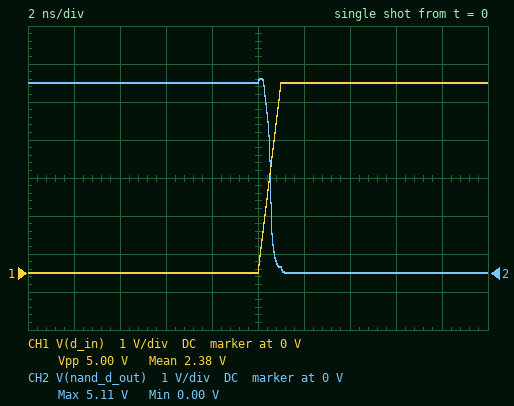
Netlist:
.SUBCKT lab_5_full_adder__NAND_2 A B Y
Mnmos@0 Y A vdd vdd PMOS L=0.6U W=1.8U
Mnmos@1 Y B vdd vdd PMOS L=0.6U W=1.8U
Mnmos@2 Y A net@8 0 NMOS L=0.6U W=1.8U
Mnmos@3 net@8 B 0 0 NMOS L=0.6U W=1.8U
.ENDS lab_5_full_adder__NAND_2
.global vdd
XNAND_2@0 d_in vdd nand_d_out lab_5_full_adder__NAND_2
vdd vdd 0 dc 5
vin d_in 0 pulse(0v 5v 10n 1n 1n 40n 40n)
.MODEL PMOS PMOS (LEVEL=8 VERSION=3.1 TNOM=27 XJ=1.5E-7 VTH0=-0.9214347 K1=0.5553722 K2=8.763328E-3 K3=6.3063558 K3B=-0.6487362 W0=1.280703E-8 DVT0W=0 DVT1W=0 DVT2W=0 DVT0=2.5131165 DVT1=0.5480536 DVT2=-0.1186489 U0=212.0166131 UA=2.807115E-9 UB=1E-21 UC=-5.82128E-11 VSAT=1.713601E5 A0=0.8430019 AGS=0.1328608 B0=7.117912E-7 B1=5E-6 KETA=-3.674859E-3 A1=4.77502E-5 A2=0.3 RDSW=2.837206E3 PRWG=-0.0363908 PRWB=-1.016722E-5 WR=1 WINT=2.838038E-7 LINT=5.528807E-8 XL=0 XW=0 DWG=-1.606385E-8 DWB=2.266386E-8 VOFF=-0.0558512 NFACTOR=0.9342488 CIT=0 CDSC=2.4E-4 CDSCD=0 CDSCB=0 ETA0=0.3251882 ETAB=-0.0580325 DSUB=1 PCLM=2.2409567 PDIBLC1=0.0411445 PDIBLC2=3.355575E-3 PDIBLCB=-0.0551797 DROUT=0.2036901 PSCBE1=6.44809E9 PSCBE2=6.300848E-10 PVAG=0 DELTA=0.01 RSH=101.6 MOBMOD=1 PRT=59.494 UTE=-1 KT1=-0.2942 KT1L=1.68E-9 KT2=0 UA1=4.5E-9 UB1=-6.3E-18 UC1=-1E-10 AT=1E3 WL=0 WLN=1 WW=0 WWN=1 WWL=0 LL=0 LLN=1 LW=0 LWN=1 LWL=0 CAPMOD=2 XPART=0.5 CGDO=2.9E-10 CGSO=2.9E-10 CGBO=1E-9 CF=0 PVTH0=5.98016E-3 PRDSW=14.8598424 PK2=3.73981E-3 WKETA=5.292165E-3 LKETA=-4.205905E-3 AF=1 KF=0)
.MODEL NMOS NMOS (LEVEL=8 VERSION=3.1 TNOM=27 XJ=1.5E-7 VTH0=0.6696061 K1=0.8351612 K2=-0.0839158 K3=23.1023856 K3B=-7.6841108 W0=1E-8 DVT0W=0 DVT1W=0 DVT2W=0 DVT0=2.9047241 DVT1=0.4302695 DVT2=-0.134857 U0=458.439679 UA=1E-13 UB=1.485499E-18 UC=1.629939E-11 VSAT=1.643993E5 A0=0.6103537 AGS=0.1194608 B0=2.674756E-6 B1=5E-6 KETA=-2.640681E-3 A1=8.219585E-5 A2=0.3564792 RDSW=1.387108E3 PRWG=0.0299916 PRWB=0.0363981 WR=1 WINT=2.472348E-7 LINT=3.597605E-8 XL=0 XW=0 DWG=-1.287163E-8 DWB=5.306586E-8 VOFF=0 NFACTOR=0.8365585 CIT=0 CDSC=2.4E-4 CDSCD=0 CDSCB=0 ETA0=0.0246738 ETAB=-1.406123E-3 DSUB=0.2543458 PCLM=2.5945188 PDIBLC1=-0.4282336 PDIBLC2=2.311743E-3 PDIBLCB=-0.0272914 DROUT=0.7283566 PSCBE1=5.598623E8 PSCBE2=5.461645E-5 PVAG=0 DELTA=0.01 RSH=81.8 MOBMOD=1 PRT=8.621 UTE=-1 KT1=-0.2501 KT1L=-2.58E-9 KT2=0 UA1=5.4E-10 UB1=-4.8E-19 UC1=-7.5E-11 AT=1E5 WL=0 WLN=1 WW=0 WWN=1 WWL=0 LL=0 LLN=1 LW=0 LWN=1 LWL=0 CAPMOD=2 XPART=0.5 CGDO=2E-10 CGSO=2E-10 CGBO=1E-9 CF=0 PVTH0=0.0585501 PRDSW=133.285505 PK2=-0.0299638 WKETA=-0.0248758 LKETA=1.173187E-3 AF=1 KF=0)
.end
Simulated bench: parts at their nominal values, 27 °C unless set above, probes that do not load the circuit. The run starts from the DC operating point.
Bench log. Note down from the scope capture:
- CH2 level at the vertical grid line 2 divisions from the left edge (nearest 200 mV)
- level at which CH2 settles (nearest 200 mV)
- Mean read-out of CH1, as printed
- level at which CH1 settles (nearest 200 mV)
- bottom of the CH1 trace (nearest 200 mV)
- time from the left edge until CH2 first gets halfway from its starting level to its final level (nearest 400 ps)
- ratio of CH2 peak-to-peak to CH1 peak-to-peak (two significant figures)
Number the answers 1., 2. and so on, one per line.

1. 5.0 V
2. 0 V
3. 2.38 V
4. 5.0 V
5. 0 V
6. 10.4 ns
7. 1.0
